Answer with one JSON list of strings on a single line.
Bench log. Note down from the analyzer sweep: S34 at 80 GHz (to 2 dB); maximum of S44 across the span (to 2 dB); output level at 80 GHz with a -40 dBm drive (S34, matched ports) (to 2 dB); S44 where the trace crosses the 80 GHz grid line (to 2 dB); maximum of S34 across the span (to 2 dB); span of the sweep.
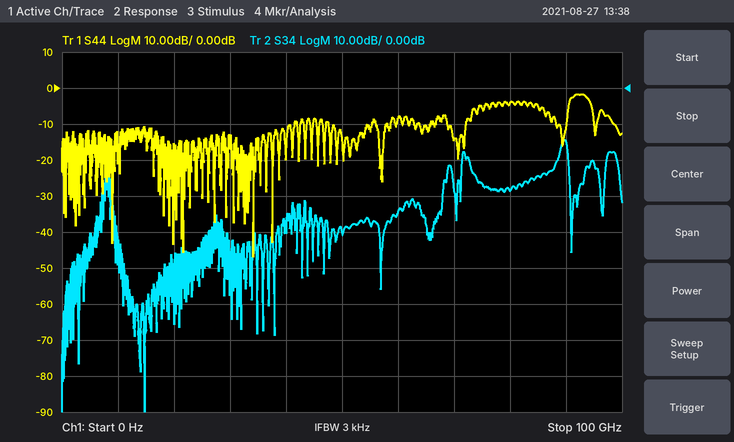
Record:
["-28 dB", "-2 dB", "-68 dBm", "-4 dB", "-14 dB", "100 GHz"]
